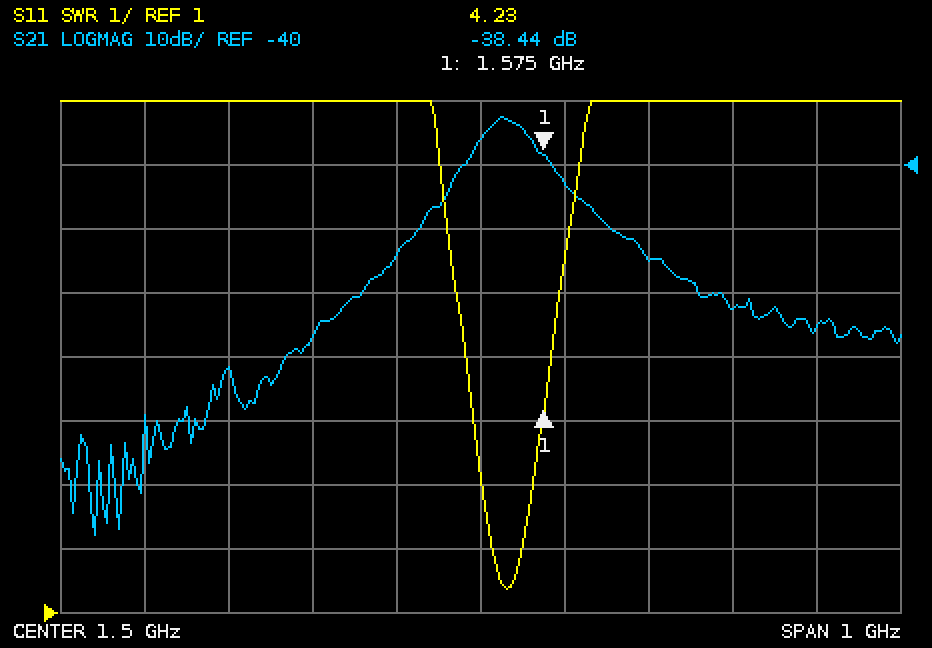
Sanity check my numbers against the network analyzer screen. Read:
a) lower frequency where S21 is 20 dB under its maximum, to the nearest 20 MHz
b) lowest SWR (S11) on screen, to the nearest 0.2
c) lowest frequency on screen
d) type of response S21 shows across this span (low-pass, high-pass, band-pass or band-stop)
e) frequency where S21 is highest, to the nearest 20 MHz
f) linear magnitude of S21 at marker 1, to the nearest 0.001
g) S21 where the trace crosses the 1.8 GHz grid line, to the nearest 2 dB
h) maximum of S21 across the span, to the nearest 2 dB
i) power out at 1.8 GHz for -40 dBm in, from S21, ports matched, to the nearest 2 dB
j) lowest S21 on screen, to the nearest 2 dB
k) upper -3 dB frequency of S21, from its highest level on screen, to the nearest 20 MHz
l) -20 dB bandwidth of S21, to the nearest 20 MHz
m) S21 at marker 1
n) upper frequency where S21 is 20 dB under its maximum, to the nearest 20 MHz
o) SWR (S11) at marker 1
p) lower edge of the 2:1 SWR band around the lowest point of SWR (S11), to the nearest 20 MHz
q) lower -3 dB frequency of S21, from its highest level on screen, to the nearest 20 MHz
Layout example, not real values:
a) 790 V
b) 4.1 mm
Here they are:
a) 1.40 GHz
b) 1.4
c) 1 GHz
d) band-pass
e) 1.52 GHz
f) 0.012
g) -62 dB
h) -32 dB
i) -102 dBm
j) -98 dB
k) 1.56 GHz
l) 280 MHz
m) -38.44 dB
n) 1.68 GHz
o) 4.23
p) 1.52 GHz
q) 1.50 GHz
